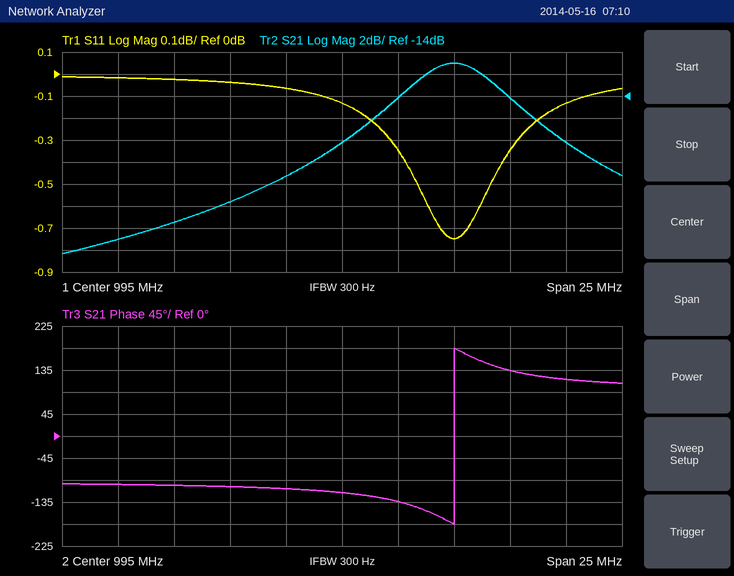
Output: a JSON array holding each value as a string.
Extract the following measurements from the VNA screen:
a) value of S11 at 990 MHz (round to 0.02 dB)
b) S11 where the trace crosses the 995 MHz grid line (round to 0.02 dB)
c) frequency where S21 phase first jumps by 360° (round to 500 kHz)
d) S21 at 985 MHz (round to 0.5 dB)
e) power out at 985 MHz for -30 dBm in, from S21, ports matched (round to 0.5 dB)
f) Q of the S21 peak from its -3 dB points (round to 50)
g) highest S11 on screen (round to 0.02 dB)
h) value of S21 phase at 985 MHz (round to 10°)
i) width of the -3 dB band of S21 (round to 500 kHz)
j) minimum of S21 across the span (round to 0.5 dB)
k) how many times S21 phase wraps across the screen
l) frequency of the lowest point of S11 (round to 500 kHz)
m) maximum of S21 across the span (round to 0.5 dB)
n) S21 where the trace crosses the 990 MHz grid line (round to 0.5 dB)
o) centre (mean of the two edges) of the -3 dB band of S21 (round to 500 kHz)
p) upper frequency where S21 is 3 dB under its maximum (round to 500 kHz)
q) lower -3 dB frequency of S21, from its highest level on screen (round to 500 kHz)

["-0.04 dB", "-0.14 dB", "1.0000 GHz", "-27.0 dB", "-57.0 dBm", "200", "-0.02 dB", "-100°", "5.0 MHz", "-28.5 dB", "1", "1.0000 GHz", "-11.0 dB", "-23.5 dB", "1.0000 GHz", "1.0025 GHz", "997.5 MHz"]
